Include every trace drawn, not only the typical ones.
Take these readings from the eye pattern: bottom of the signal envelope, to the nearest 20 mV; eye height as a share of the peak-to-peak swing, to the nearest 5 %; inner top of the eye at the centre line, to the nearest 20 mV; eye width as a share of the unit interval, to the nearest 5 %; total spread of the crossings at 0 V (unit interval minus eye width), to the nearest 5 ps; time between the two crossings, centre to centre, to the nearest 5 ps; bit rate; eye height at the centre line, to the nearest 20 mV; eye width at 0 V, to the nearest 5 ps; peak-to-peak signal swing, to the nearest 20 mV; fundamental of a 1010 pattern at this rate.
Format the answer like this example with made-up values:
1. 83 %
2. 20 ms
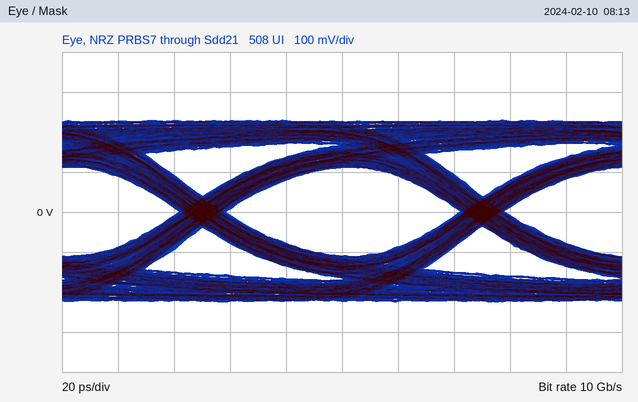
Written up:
1. -220 mV
2. 50 %
3. 120 mV
4. 85 %
5. 15 ps
6. 100 ps
7. 10 Gb/s
8. 220 mV
9. 85 ps
10. 460 mV
11. 5 GHz
